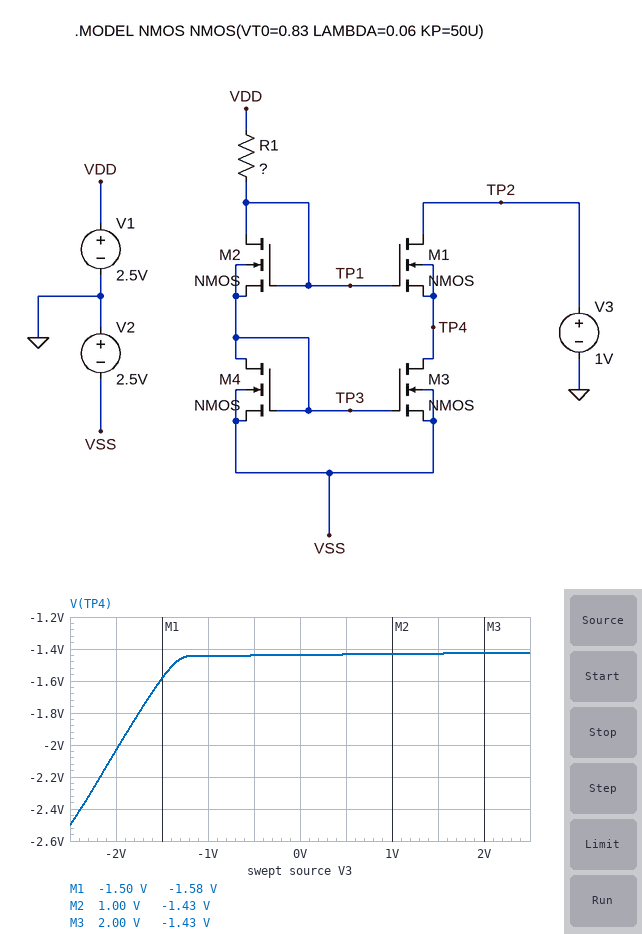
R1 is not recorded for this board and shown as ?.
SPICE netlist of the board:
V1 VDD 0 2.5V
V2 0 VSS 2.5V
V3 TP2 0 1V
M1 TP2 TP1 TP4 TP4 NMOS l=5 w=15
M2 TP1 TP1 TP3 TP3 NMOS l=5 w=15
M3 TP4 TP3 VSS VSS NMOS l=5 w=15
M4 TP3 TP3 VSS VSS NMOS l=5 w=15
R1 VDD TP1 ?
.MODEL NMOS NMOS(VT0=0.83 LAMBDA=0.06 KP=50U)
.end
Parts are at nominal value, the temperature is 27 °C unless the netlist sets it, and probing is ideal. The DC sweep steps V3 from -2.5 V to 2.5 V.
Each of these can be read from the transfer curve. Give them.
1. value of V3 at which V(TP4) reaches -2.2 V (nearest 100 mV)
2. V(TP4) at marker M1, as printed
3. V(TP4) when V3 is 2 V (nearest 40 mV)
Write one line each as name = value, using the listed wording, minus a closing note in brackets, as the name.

value of V3 at which V(TP4) reaches -2.2 V = -2.2 V
V(TP4) at marker M1, as printed = -1.58 V
V(TP4) when V3 is 2 V = -1.44 V
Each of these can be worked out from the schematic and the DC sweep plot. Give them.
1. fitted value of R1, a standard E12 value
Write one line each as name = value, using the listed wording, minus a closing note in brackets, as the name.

fitted value of R1, a standard E12 value = 680 kΩ
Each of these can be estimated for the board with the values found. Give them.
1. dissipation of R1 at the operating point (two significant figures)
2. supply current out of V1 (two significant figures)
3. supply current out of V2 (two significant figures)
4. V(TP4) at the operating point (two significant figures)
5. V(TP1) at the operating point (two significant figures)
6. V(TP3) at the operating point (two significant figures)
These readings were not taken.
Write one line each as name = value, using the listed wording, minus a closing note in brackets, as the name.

dissipation of R1 at the operating point = 12 µW
supply current out of V1 = 4.2 µA
supply current out of V2 = 8.5 µA
V(TP4) at the operating point = -1.4 V
V(TP1) at the operating point = -380 mV
V(TP3) at the operating point = -1.4 V
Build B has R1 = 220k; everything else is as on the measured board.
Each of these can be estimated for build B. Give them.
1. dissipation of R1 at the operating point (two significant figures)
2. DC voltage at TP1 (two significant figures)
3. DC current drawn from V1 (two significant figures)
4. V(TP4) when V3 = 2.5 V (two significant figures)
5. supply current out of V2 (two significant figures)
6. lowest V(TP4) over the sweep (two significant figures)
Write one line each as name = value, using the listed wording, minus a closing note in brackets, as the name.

dissipation of R1 at the operating point = 30 µW
DC voltage at TP1 = -77 mV
DC current drawn from V1 = 12 µA
V(TP4) when V3 = 2.5 V = -1.3 V
supply current out of V2 = 23 µA
lowest V(TP4) over the sweep = -2.5 V
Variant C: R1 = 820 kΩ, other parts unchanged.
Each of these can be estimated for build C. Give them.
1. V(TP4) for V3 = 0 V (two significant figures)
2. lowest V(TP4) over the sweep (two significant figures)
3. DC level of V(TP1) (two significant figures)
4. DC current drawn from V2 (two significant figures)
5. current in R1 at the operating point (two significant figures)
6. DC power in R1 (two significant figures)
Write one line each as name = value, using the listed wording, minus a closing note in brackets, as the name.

V(TP4) for V3 = 0 V = -1.5 V
lowest V(TP4) over the sweep = -2.5 V
DC level of V(TP1) = -420 mV
DC current drawn from V2 = 7.1 µA
current in R1 at the operating point = 3.6 µA
DC power in R1 = 10 µW
